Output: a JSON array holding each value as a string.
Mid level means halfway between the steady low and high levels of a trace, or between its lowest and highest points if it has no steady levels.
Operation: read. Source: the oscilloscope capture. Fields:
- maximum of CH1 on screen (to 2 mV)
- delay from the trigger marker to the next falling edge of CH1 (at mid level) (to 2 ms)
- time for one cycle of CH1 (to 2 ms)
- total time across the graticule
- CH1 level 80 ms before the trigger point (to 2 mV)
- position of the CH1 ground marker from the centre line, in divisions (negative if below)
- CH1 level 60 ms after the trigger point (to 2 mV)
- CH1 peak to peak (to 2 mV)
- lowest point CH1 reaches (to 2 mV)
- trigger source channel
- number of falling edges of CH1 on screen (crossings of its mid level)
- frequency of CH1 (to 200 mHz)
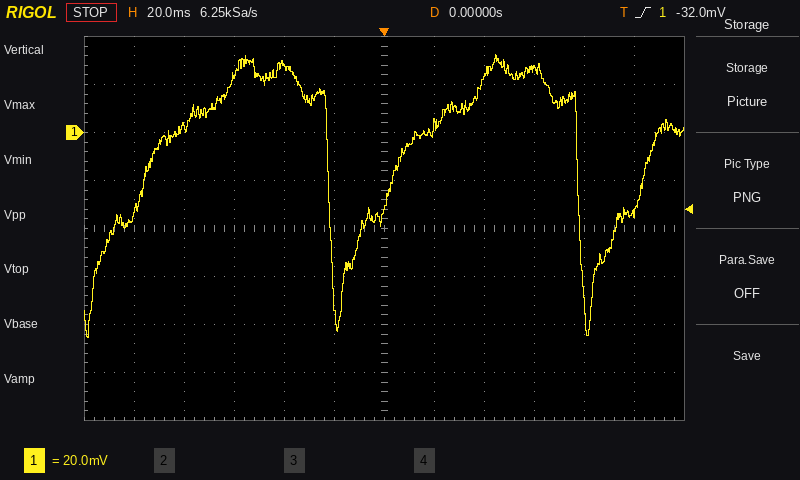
["32 mV", "78 ms", "100 ms", "240 ms", "2 mV", "+2.0 div", "26 mV", "118 mV", "-86 mV", "CH1", "2", "10.0 Hz"]
